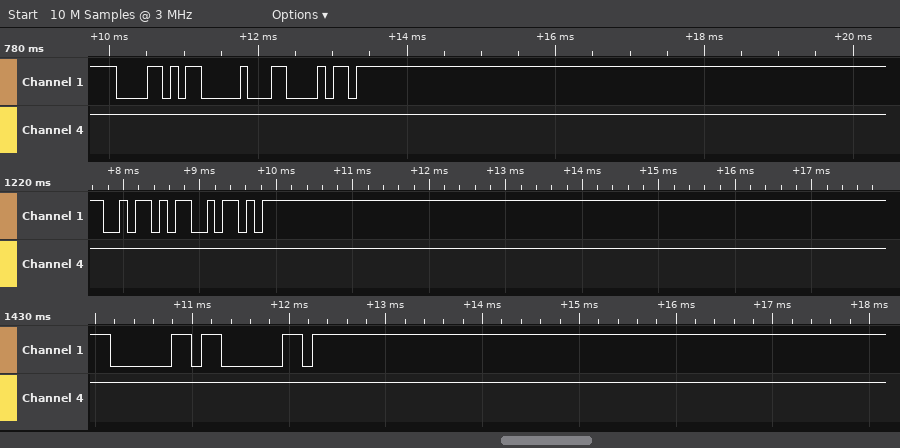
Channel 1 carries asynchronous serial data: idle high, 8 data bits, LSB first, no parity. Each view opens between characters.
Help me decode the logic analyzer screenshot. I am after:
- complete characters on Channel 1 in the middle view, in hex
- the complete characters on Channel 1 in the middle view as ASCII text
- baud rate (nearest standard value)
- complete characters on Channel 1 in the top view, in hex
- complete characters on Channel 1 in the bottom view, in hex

5A, 5A
"ZZ"
9600 baud
58, 10, 68
60, 60
